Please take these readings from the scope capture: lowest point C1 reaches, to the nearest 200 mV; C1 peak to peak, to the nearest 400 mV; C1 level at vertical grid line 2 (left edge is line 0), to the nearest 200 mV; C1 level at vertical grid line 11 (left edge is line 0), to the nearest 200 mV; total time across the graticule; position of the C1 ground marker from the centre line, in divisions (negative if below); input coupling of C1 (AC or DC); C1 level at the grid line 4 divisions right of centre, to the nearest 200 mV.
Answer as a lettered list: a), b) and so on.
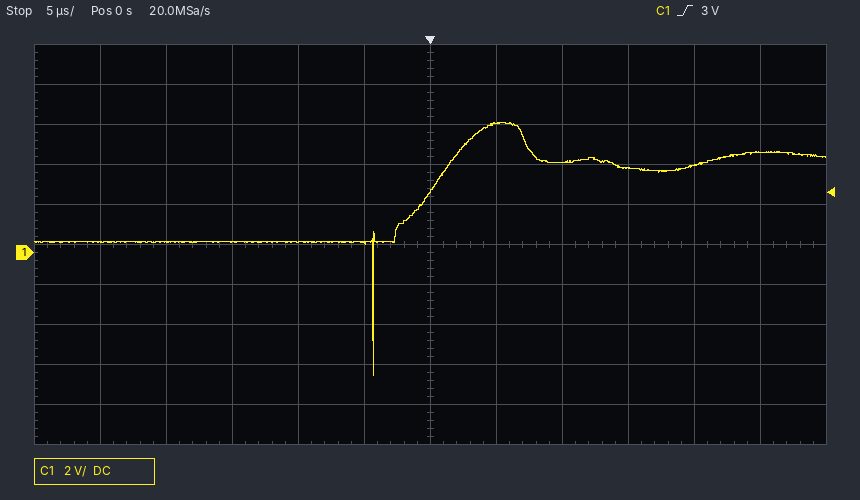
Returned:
a) -6.2 V
b) 12.8 V
c) 600 mV
d) 5.0 V
e) 60 µs
f) -0.2 div
g) DC
h) 4.4 V
